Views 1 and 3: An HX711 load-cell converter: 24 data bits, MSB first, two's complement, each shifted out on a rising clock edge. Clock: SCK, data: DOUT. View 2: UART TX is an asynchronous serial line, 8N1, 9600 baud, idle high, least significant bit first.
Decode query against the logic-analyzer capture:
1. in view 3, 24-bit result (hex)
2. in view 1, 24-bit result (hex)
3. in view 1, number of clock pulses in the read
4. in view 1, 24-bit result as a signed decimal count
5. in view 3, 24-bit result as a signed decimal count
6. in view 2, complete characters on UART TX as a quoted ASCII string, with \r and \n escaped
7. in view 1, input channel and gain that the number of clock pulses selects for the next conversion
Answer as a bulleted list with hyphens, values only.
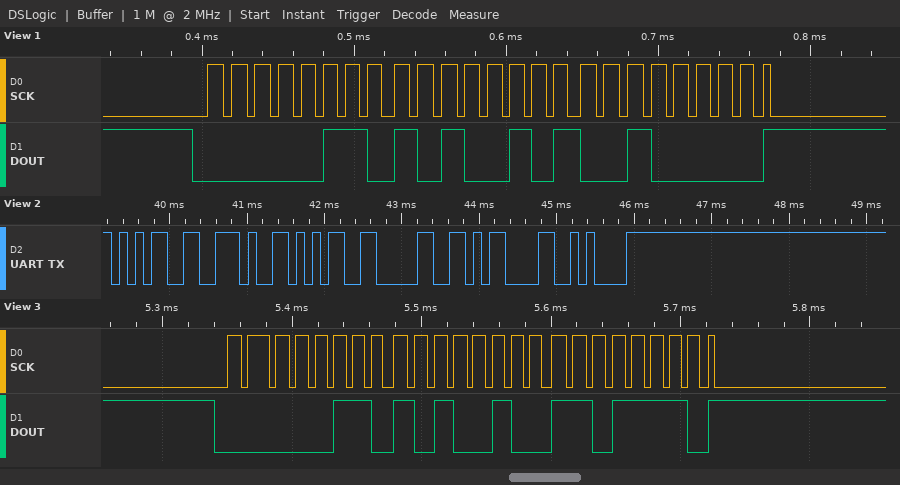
- 0x06A4DE
- 0x06A520
- 25
- 435488
- 435422
- "5.50\r\n"
- channel A, gain 128
